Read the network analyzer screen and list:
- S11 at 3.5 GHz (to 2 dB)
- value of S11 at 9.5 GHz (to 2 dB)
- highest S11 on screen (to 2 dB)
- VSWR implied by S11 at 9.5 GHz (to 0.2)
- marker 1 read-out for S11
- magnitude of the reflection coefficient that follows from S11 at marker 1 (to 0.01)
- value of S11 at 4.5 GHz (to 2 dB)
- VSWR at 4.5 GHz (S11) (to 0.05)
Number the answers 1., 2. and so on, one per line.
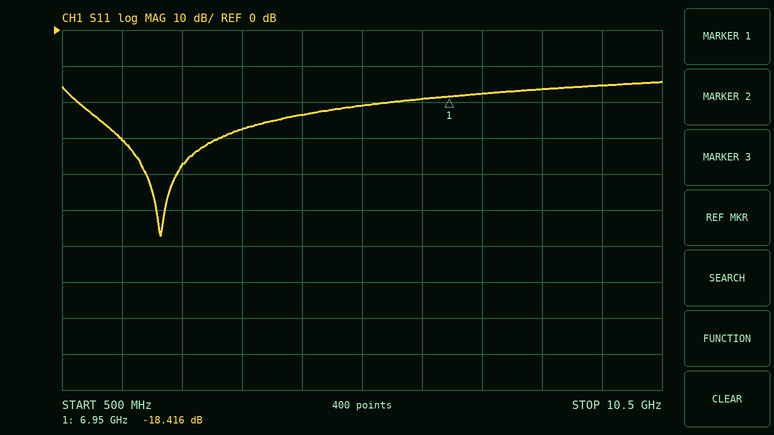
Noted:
1. -28 dB
2. -16 dB
3. -14 dB
4. 1.4
5. -18.416 dB
6. 0.12
7. -24 dB
8. 1.15
